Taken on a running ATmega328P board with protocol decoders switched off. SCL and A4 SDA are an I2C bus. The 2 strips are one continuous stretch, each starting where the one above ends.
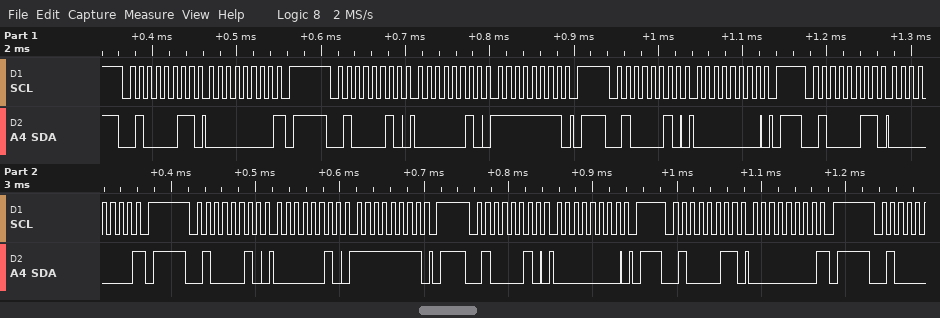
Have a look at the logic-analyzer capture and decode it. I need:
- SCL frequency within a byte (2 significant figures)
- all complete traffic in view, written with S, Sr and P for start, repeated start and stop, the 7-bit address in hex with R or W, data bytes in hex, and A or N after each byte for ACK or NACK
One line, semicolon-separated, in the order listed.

100 kHz; S 21R A 00 N P S 21W A 02 A FF A P S 21W A 00 A P S 21R A 00 N P S 21W A 02 A FF A P S 21W A 00 A P S 21R A 00 N P
